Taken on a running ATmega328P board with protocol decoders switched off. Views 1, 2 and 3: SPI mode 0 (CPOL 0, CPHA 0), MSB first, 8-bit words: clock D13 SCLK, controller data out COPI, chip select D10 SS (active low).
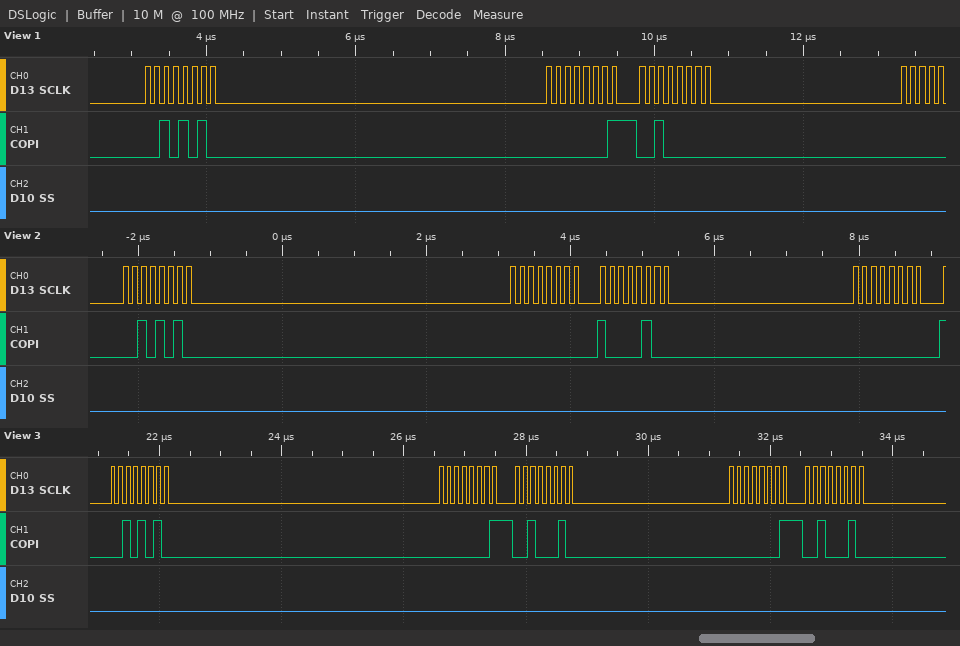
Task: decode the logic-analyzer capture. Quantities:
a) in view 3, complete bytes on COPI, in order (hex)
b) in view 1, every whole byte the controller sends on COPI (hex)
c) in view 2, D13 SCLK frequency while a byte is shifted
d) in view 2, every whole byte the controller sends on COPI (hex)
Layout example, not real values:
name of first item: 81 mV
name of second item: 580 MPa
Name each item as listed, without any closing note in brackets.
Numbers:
in view 3, complete bytes on COPI, in order: 0x2A 0x01 0x22 0x01 0x22
in view 1, every whole byte the controller sends on COPI: 2A 01 20
in view 2, D13 SCLK frequency while a byte is shifted: 8 MHz
in view 2, every whole byte the controller sends on COPI: 2A 00 84 00
